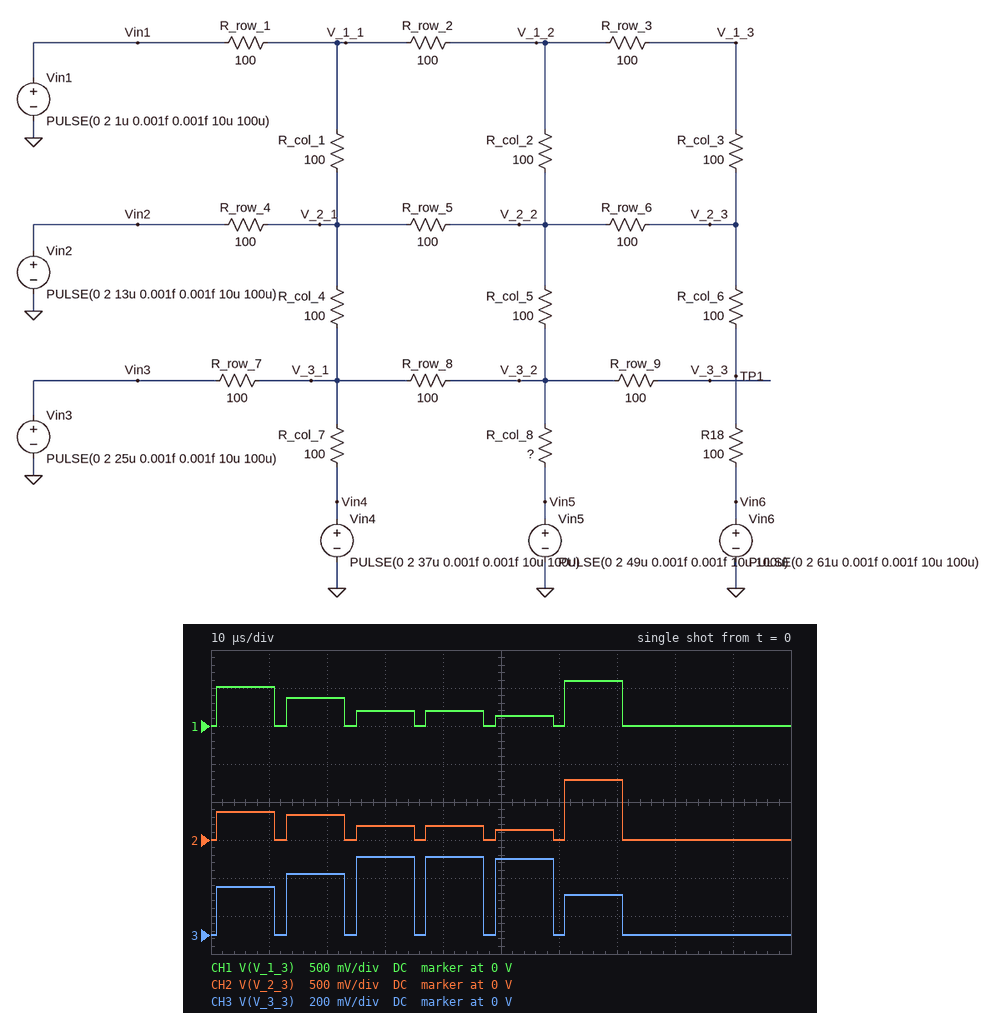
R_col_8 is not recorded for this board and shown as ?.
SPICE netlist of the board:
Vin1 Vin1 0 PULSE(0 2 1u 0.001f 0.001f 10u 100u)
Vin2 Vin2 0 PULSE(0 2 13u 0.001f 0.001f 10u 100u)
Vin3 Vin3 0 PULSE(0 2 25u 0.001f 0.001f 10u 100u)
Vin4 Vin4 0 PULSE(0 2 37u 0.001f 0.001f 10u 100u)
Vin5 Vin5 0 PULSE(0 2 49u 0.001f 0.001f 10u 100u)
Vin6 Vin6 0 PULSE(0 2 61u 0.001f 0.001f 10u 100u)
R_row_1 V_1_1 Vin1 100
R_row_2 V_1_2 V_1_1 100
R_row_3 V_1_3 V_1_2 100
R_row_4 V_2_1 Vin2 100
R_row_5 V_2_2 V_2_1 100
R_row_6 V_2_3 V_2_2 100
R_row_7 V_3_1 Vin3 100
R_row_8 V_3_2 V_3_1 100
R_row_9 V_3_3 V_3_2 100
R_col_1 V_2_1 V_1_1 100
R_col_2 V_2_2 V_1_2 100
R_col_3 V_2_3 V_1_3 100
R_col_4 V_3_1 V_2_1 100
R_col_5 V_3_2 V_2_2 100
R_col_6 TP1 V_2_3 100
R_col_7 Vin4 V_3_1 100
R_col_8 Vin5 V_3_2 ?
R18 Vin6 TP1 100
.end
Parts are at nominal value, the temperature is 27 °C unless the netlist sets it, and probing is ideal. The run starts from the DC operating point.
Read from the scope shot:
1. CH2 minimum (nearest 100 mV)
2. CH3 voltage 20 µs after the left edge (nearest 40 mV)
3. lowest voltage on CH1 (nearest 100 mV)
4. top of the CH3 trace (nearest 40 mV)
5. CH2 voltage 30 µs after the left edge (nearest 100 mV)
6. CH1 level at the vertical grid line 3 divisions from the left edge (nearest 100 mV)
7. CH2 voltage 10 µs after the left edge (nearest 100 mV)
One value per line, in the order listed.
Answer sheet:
0 V
320 mV
0 V
400 mV
200 mV
200 mV
400 mV
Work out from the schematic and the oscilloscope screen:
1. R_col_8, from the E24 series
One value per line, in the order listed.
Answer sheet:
330 Ω
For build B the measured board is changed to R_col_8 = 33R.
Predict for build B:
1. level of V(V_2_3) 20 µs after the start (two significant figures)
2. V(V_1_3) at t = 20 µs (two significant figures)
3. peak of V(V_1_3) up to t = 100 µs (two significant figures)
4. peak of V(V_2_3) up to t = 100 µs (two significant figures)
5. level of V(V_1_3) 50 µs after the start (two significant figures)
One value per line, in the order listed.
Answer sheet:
270 mV
310 mV
550 mV
750 mV
460 mV
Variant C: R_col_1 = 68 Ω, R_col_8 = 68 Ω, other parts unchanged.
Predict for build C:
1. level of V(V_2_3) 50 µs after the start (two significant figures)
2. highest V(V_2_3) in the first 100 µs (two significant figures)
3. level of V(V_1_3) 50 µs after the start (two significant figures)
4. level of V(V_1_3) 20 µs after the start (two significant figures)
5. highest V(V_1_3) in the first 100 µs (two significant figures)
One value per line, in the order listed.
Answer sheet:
350 mV
760 mV
360 mV
340 mV
560 mV
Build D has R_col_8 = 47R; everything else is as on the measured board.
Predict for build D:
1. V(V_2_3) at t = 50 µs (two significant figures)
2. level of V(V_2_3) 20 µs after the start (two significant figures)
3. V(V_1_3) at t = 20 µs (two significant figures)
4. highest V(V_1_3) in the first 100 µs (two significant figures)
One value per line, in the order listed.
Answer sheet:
410 mV
280 mV
320 mV
550 mV
